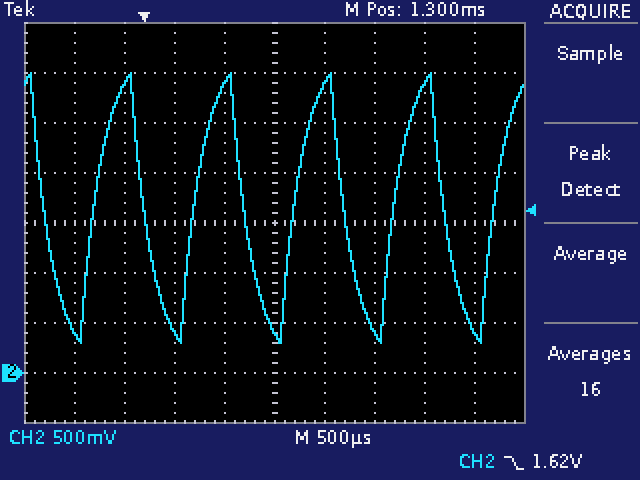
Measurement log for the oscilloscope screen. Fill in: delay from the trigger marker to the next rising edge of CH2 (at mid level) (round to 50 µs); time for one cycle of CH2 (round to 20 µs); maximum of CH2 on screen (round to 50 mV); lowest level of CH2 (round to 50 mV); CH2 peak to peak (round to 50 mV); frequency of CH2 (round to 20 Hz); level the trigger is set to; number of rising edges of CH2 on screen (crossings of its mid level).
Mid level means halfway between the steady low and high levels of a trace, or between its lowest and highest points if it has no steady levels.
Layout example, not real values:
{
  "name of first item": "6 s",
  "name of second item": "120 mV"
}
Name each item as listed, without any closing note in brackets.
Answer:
{
  "delay from the trigger marker to the next rising edge of CH2 (at mid level)": "500 µs",
  "time for one cycle of CH2": "1.00 ms",
  "maximum of CH2 on screen": "3.00 V",
  "lowest level of CH2": "300 mV",
  "CH2 peak to peak": "2.70 V",
  "frequency of CH2": "1.00 kHz",
  "level the trigger is set to": "1.62 V",
  "number of rising edges of CH2 on screen": "5"
}
